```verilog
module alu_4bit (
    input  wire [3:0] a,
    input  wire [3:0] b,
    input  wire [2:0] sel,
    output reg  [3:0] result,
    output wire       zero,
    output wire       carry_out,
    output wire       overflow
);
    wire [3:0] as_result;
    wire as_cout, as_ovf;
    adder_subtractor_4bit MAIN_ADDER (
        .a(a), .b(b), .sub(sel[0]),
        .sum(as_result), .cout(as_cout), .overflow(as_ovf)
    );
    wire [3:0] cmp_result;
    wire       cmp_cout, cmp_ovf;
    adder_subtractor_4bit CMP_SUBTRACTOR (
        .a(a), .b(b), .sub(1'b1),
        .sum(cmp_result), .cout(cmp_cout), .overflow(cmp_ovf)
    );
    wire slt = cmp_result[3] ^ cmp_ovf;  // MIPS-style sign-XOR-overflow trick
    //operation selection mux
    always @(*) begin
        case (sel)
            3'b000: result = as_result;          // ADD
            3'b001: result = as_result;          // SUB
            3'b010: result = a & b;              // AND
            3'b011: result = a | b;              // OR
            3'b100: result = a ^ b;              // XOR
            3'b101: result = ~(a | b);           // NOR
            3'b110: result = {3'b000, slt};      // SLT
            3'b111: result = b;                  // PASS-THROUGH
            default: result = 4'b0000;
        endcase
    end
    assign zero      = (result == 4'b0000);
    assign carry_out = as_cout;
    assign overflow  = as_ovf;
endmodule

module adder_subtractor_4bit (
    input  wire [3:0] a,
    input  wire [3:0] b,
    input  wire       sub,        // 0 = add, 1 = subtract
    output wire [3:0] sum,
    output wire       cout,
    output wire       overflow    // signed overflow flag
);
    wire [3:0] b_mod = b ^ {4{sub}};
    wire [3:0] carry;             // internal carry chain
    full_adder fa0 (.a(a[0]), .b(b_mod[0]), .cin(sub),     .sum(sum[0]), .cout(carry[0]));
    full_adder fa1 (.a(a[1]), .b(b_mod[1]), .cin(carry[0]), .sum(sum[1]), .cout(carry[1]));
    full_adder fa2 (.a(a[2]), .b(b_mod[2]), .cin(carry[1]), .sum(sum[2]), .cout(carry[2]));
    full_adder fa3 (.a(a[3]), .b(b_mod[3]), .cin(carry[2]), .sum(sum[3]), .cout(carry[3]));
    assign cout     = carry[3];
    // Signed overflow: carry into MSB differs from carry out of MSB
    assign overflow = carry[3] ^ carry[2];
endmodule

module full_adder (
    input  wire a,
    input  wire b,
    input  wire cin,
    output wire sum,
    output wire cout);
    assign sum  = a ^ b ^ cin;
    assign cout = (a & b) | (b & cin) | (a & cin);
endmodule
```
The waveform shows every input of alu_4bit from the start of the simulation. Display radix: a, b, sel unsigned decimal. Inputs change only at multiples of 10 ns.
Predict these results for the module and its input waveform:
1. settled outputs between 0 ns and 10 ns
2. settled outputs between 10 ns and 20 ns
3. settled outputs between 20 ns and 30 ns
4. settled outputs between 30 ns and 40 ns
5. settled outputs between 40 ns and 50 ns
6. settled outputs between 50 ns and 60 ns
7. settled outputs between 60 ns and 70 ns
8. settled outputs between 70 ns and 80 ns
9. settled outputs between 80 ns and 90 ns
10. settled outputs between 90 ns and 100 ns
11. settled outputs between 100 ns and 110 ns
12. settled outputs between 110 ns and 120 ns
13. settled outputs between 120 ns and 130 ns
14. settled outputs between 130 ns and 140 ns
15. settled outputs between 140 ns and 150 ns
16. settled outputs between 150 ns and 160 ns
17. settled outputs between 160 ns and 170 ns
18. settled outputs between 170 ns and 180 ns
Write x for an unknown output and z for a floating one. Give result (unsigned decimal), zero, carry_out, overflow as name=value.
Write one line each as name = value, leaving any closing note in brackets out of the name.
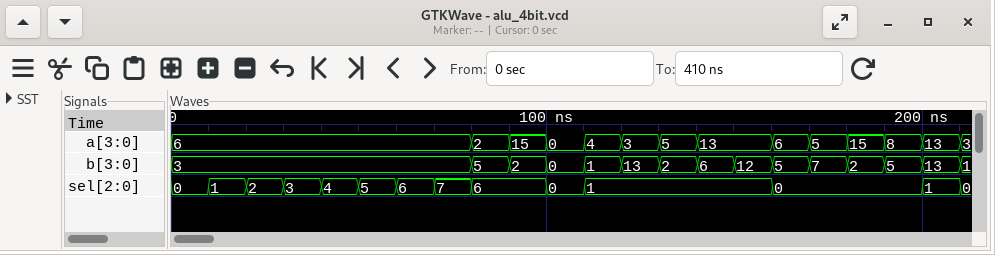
settled outputs between 0 ns and 10 ns = result=9, zero=0, carry_out=0, overflow=1
settled outputs between 10 ns and 20 ns = result=3, zero=0, carry_out=1, overflow=0
settled outputs between 20 ns and 30 ns = result=2, zero=0, carry_out=0, overflow=1
settled outputs between 30 ns and 40 ns = result=7, zero=0, carry_out=1, overflow=0
settled outputs between 40 ns and 50 ns = result=5, zero=0, carry_out=0, overflow=1
settled outputs between 50 ns and 60 ns = result=8, zero=0, carry_out=1, overflow=0
settled outputs between 60 ns and 70 ns = result=0, zero=1, carry_out=0, overflow=1
settled outputs between 70 ns and 80 ns = result=3, zero=0, carry_out=1, overflow=0
settled outputs between 80 ns and 90 ns = result=1, zero=0, carry_out=0, overflow=0
settled outputs between 90 ns and 100 ns = result=1, zero=0, carry_out=1, overflow=0
settled outputs between 100 ns and 110 ns = result=0, zero=1, carry_out=0, overflow=0
settled outputs between 110 ns and 120 ns = result=3, zero=0, carry_out=1, overflow=0
settled outputs between 120 ns and 130 ns = result=6, zero=0, carry_out=0, overflow=0
settled outputs between 130 ns and 140 ns = result=3, zero=0, carry_out=1, overflow=0
settled outputs between 140 ns and 150 ns = result=7, zero=0, carry_out=1, overflow=1
settled outputs between 150 ns and 160 ns = result=1, zero=0, carry_out=1, overflow=0
settled outputs between 160 ns and 170 ns = result=11, zero=0, carry_out=0, overflow=1
settled outputs between 170 ns and 180 ns = result=12, zero=0, carry_out=0, overflow=1
